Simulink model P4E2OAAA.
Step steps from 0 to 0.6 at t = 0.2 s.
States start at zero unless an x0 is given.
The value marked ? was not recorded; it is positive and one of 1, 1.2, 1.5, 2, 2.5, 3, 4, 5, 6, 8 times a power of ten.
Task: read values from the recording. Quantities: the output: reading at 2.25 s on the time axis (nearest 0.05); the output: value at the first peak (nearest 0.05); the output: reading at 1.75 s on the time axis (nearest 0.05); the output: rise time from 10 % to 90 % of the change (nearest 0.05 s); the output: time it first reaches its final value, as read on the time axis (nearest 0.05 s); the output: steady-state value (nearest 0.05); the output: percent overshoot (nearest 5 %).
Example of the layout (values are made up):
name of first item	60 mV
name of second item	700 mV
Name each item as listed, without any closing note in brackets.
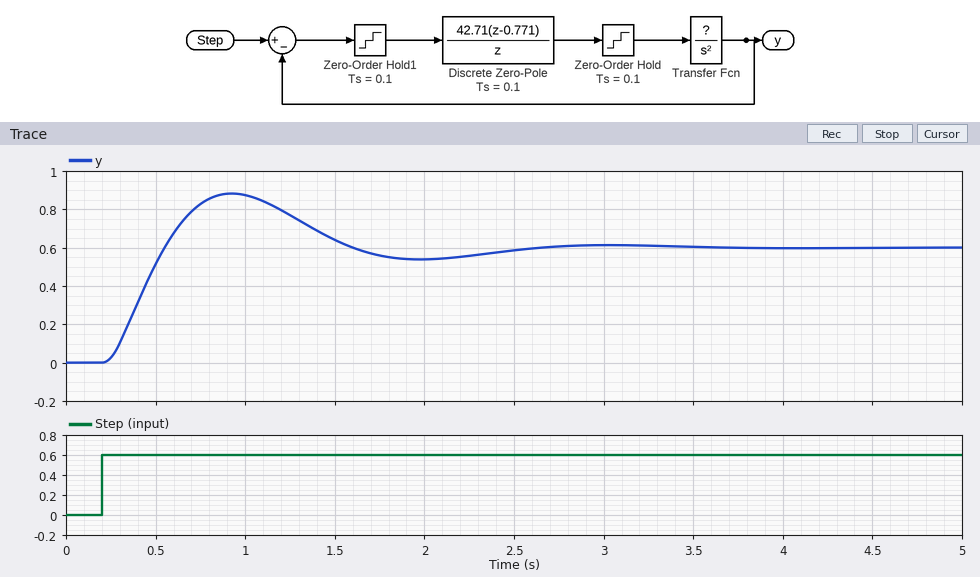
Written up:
the output: reading at 2.25 s on the time axis	0.55
the output: value at the first peak	0.90
the output: reading at 1.75 s on the time axis	0.55
the output: rise time from 10 % to 90 % of the change	0.25 s
the output: time it first reaches its final value, as read on the time axis	0.55 s
the output: steady-state value	0.60
the output: percent overshoot	45 %
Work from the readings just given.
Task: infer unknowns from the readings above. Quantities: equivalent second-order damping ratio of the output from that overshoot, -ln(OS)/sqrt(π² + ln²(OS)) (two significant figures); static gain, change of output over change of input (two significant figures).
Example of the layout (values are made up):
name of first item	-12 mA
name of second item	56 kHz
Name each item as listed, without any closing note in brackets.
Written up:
equivalent second-order damping ratio of the output from that overshoot, -ln(OS)/sqrt(π² + ln²(OS))	0.25
static gain, change of output over change of input	1.0
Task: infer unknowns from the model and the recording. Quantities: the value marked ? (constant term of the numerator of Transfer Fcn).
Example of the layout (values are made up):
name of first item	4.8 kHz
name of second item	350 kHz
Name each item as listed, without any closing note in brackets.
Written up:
the value marked ?	0.8
